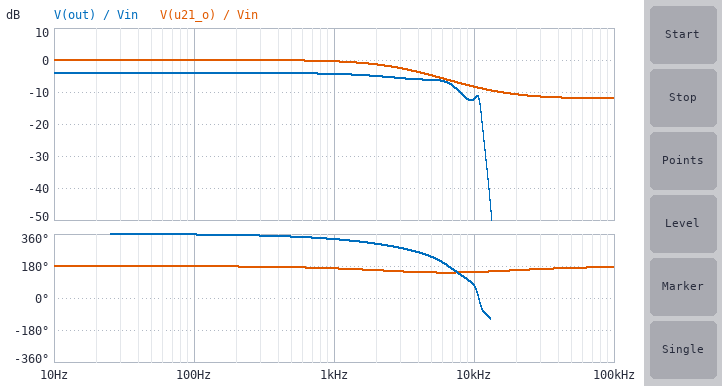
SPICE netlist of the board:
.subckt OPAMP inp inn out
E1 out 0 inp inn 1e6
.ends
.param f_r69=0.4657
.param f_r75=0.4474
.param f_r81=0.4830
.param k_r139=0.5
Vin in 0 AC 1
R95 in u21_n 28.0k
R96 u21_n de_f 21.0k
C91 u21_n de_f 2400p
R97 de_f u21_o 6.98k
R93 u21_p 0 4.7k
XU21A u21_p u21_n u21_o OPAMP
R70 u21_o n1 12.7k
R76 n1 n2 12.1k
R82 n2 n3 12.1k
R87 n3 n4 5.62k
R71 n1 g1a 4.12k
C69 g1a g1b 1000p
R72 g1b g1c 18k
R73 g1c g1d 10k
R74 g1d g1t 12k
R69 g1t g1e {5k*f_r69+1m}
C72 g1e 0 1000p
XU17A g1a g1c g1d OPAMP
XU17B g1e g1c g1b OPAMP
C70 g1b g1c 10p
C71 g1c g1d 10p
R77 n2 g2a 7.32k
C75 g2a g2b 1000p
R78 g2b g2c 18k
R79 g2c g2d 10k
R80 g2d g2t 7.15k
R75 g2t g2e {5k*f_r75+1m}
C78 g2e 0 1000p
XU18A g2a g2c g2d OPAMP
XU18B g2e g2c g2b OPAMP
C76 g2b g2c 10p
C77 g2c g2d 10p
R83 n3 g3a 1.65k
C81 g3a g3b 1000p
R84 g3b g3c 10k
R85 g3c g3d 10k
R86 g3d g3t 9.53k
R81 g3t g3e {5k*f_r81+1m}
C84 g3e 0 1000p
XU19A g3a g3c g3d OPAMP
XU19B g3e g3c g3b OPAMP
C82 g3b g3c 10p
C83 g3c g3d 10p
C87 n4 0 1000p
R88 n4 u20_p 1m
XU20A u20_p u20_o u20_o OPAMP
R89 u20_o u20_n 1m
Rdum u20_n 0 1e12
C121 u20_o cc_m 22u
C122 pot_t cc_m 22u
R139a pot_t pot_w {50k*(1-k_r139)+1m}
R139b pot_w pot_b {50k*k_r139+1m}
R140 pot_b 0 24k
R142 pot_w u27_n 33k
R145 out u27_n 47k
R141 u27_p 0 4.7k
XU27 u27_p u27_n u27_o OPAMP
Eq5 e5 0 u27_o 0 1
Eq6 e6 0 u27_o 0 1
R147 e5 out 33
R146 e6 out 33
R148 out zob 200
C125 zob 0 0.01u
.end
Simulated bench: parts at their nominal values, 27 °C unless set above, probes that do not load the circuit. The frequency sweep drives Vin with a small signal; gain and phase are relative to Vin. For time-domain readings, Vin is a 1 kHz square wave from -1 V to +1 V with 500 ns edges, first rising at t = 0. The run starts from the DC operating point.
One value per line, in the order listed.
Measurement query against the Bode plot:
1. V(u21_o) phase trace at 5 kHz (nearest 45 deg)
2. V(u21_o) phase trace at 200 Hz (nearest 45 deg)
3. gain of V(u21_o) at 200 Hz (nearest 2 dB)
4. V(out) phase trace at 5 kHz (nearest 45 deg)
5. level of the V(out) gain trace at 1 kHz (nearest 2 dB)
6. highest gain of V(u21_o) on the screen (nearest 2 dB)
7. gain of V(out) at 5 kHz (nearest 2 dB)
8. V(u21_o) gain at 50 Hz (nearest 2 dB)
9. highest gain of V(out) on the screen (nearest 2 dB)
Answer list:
135 deg
180 deg
0 dB
225 deg
-4 dB
0 dB
-6 dB
0 dB
-4 dB
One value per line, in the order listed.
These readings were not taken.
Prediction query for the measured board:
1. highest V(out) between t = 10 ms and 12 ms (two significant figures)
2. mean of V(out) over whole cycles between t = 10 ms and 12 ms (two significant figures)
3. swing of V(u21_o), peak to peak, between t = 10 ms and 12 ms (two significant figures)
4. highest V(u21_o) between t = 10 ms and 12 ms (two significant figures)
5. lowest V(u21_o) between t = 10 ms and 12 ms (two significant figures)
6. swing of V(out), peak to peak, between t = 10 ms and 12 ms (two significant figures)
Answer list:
1.3 V
610 mV
2.0 V
1.0 V
-1.0 V
1.3 V
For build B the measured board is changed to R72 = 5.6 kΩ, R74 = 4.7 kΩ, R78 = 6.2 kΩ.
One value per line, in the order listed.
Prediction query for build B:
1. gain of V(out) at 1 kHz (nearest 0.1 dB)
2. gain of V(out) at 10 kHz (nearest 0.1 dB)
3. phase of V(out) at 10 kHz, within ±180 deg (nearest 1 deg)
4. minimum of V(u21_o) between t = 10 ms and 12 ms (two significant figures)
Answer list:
-4.5 dB
-16.3 dB
-167 deg
-1.0 V
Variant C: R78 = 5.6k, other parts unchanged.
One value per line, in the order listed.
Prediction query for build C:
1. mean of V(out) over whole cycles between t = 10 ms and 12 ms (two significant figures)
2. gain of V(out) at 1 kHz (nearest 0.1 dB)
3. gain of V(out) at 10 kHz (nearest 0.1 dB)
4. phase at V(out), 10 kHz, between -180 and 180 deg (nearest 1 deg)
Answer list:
610 mV
-4.4 dB
-14.0 dB
73 deg
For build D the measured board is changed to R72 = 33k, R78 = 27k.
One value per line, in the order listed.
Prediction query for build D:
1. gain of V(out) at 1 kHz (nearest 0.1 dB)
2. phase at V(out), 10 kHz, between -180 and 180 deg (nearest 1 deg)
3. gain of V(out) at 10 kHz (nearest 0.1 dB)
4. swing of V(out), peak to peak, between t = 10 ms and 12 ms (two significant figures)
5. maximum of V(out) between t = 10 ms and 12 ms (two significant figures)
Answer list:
-4.2 dB
-79 deg
-40.7 dB
1.7 V
1.5 V
